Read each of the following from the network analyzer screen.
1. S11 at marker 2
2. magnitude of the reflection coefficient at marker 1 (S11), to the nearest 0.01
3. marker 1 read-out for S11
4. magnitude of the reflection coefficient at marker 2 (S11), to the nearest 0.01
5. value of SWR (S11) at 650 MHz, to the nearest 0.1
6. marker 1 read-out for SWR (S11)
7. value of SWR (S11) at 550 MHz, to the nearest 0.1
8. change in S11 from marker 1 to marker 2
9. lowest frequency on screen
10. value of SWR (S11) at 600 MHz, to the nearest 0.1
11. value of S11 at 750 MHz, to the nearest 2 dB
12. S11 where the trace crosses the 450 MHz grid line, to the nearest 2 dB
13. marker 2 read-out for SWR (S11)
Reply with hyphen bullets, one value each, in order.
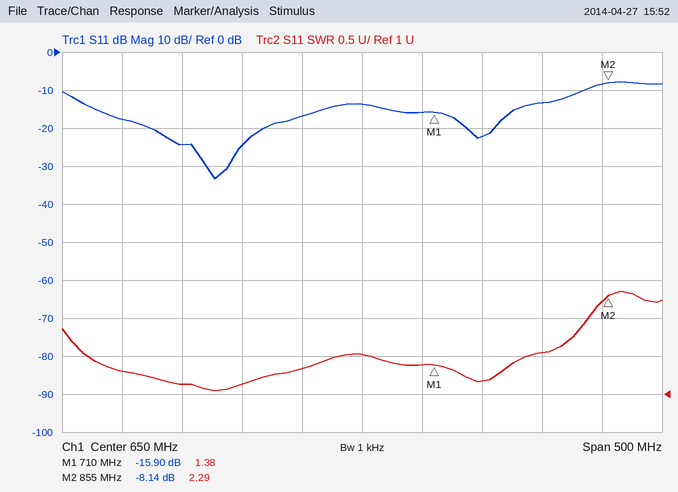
- -8.14 dB
- 0.16
- -15.90 dB
- 0.39
- 1.5
- 1.38
- 1.1
- 7.76 dB
- 400 MHz
- 1.3
- -22 dB
- -18 dB
- 2.29
